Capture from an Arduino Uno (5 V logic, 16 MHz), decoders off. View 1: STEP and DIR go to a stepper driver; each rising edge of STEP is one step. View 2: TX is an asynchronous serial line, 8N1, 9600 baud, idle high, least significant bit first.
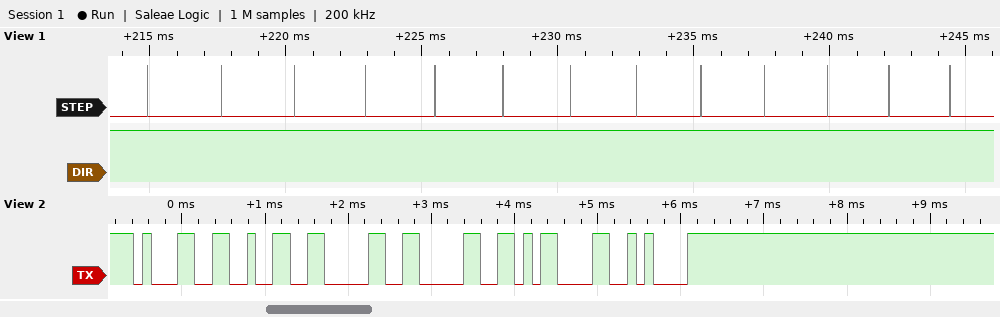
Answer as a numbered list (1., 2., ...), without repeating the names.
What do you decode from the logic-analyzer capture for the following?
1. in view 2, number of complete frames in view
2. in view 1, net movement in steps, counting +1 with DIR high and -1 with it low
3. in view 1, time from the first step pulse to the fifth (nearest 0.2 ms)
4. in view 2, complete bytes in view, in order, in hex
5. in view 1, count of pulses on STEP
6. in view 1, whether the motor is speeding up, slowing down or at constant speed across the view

1. 6
2. +13
3. 10.6 ms
4. 31 32 30 30 0D 0A
5. 13
6. speeding up
